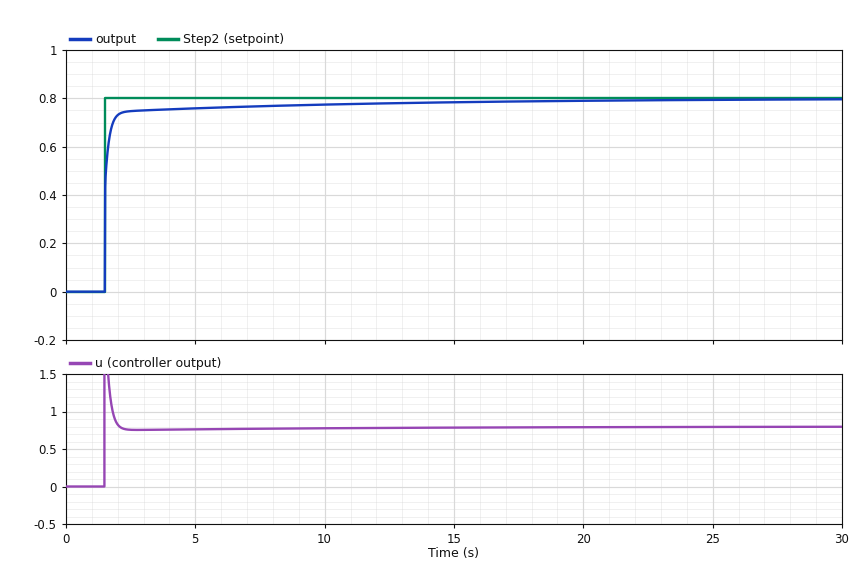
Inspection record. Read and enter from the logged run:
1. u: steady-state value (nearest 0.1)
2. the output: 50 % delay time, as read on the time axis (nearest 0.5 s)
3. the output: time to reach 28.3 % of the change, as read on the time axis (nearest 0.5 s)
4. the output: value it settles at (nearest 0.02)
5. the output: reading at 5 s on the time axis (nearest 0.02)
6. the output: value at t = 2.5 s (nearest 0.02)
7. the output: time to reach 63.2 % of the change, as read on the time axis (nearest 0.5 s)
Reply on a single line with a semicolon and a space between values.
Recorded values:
0.8; 1.5 s; 1.5 s; 0.80; 0.76; 0.74; 1.5 s
